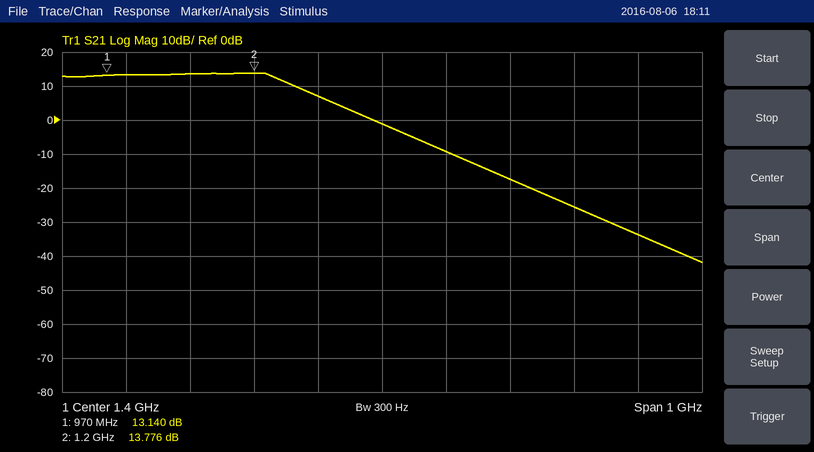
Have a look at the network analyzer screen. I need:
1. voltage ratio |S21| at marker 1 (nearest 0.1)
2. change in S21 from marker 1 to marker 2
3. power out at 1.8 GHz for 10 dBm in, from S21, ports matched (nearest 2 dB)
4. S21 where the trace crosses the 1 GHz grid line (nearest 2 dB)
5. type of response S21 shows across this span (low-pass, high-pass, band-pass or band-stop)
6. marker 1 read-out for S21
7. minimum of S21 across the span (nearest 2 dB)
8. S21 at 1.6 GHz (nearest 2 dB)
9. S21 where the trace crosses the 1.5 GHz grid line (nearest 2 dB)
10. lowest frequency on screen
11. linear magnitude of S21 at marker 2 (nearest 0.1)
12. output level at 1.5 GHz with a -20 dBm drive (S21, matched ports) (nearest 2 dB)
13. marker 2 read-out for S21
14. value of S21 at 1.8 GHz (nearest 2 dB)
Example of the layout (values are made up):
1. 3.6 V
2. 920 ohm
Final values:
1. 4.5
2. 0.636 dB
3. -24 dBm
4. 14 dB
5. low-pass
6. 13.140 dB
7. -42 dB
8. -18 dB
9. -10 dB
10. 900 MHz
11. 4.9
12. -30 dBm
13. 13.776 dB
14. -34 dB
